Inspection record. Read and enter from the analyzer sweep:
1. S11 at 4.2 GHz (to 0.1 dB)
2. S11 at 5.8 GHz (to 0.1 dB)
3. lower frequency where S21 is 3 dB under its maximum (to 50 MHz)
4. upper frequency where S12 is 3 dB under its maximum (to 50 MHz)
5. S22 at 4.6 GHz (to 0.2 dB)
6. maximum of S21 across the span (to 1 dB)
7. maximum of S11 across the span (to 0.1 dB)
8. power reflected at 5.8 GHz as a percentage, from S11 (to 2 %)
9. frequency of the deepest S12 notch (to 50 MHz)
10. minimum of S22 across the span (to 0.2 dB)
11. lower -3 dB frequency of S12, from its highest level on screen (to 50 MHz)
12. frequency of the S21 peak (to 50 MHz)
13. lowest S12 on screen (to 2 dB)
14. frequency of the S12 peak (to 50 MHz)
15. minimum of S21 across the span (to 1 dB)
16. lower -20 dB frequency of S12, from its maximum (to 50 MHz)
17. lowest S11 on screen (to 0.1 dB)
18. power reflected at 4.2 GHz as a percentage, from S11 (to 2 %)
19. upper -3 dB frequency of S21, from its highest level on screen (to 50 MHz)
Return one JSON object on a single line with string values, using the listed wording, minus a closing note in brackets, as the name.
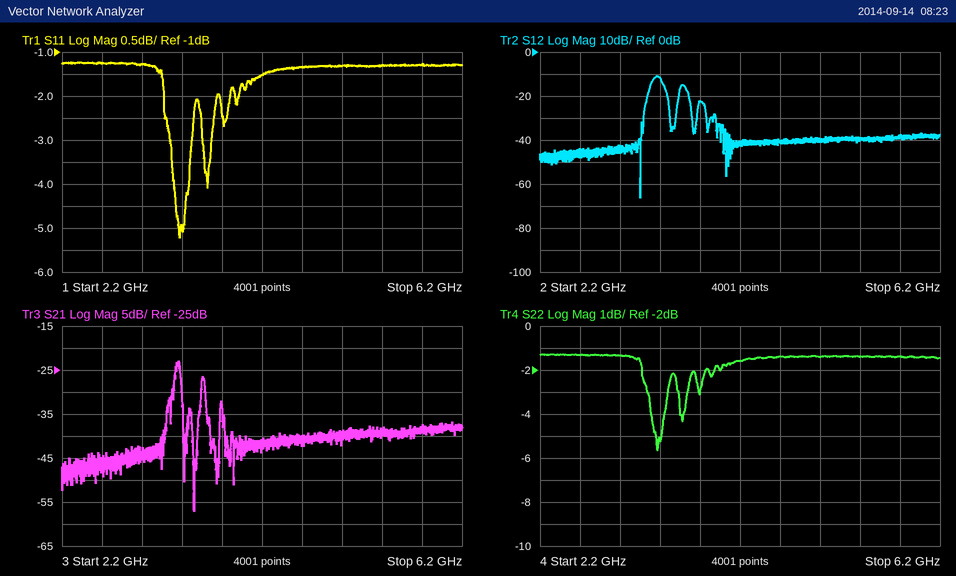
{"S11 at 4.2 GHz": "-1.5 dB", "S11 at 5.8 GHz": "-1.3 dB", "lower frequency where S21 is 3 dB under its maximum": "3.35 GHz", "upper frequency where S12 is 3 dB under its maximum": "3.40 GHz", "S22 at 4.6 GHz": "-1.4 dB", "maximum of S21 across the span": "-23 dB", "maximum of S11 across the span": "-1.2 dB", "power reflected at 5.8 GHz as a percentage, from S11": "74 %", "frequency of the deepest S12 notch": "3.20 GHz", "minimum of S22 across the span": "-5.6 dB", "lower -3 dB frequency of S12, from its highest level on screen": "3.30 GHz", "frequency of the S21 peak": "3.35 GHz", "lowest S12 on screen": "-66 dB", "frequency of the S12 peak": "3.35 GHz", "minimum of S21 across the span": "-57 dB", "lower -20 dB frequency of S12, from its maximum": "3.25 GHz", "lowest S11 on screen": "-5.2 dB", "power reflected at 4.2 GHz as a percentage, from S11": "70 %", "upper -3 dB frequency of S21, from its highest level on screen": "3.40 GHz"}
